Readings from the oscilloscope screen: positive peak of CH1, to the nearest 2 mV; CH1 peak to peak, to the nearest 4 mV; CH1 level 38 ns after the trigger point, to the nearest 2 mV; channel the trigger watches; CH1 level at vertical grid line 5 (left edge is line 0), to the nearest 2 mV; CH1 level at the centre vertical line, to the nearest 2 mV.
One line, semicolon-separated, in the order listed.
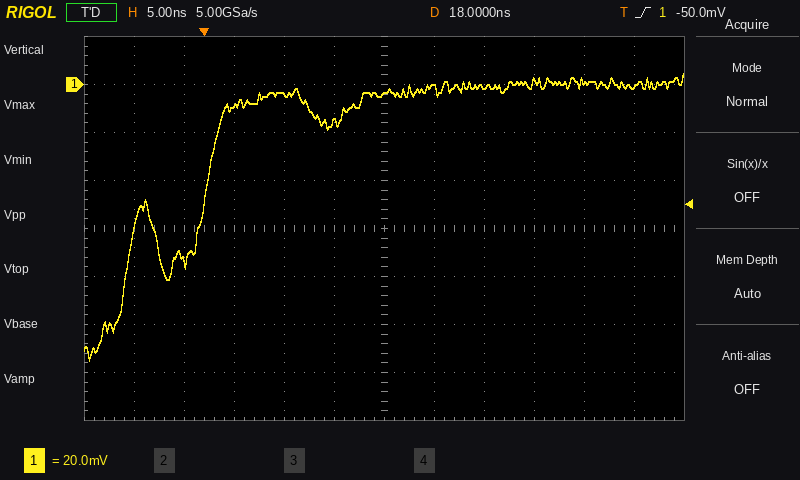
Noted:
4 mV; 120 mV; 2 mV; CH1; -16 mV; -4 mV
